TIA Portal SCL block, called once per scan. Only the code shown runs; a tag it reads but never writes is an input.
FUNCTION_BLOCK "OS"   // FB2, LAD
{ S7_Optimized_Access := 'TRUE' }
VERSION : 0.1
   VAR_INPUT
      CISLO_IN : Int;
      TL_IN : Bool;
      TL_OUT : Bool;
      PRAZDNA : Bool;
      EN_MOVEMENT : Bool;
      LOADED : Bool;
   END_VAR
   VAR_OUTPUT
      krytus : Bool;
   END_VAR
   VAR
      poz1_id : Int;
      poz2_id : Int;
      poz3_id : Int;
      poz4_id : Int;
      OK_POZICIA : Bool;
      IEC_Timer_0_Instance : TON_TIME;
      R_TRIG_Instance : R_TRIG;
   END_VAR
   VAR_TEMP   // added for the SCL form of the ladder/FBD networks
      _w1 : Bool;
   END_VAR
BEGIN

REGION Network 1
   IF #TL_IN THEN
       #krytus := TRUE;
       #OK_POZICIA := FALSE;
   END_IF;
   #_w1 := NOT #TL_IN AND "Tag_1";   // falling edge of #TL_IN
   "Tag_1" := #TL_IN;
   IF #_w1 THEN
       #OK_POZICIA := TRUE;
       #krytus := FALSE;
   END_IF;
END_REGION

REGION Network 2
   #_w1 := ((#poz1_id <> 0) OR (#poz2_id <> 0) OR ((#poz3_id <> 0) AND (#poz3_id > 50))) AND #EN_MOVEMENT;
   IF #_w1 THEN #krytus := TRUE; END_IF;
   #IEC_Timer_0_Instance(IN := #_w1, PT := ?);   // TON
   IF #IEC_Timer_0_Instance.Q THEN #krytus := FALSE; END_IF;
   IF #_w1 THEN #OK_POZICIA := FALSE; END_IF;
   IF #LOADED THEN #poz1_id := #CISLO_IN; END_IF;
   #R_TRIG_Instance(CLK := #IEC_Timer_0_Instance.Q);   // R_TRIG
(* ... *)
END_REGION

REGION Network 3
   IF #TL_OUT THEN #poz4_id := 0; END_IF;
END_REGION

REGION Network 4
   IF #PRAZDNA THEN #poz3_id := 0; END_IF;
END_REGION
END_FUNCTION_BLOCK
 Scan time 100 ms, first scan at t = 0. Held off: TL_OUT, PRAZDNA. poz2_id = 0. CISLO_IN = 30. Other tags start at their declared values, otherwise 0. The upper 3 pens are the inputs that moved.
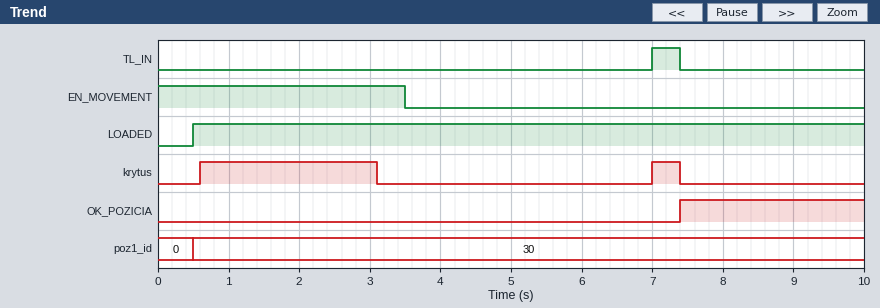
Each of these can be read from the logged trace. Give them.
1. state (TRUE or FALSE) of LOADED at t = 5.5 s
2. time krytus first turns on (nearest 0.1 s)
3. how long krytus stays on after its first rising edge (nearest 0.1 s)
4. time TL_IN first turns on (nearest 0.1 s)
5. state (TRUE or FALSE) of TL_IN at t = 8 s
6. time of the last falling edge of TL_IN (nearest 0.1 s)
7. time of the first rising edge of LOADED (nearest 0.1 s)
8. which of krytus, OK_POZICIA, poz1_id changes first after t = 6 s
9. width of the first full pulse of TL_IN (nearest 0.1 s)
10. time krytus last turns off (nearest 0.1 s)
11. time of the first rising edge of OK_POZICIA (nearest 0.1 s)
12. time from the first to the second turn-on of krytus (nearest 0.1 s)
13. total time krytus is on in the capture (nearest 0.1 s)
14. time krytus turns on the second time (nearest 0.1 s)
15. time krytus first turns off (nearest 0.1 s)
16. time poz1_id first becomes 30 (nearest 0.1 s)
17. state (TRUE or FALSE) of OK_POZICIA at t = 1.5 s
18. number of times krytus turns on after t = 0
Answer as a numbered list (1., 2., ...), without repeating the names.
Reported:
1. TRUE
2. 0.6 s
3. 2.5 s
4. 7.0 s
5. FALSE
6. 7.4 s
7. 0.5 s
8. krytus
9. 0.4 s
10. 7.4 s
11. 7.4 s
12. 6.4 s
13. 2.9 s
14. 7.0 s
15. 3.1 s
16. 0.5 s
17. FALSE
18. 2
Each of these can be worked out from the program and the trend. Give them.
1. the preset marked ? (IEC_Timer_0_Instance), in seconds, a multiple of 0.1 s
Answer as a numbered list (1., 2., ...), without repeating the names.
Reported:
1. 2.5 s
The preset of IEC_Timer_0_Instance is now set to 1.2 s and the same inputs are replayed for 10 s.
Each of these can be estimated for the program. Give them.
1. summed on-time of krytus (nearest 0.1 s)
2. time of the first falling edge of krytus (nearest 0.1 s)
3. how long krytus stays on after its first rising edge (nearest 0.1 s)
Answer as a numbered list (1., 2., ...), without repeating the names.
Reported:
1. 1.6 s
2. 1.8 s
3. 1.2 s
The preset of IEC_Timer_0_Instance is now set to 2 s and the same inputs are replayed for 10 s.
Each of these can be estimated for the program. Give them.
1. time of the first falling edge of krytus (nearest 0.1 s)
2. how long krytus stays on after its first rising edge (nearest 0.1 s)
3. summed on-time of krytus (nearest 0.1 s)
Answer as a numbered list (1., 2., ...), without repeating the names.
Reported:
1. 2.6 s
2. 2.0 s
3. 2.4 s
